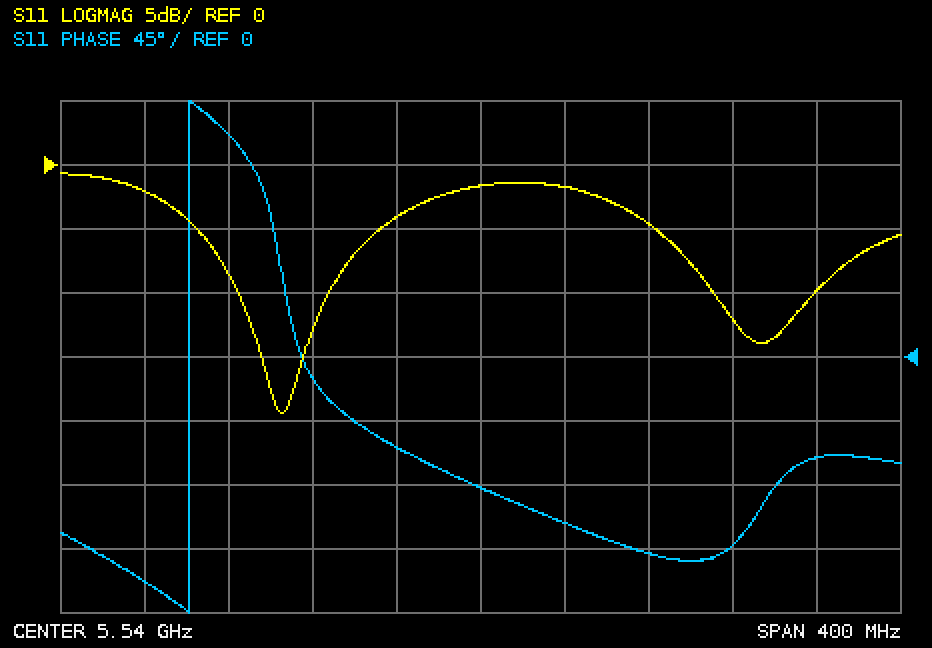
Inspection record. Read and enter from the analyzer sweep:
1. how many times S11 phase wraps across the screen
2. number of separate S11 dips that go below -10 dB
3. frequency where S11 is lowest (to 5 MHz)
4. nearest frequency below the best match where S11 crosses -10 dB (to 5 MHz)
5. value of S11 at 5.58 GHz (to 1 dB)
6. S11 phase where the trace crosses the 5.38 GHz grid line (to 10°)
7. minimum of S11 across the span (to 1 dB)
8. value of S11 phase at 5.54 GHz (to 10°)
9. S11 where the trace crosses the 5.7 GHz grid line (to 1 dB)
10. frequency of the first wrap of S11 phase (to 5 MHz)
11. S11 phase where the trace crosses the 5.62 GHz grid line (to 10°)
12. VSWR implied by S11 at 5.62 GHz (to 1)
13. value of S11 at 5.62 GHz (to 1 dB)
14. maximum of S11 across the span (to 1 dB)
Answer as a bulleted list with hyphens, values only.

- 1
- 2
- 5.445 GHz
- 5.425 GHz
- -2 dB
- -160°
- -19 dB
- -90°
- -10 dB
- 5.400 GHz
- -140°
- 4
- -5 dB
- -1 dB
